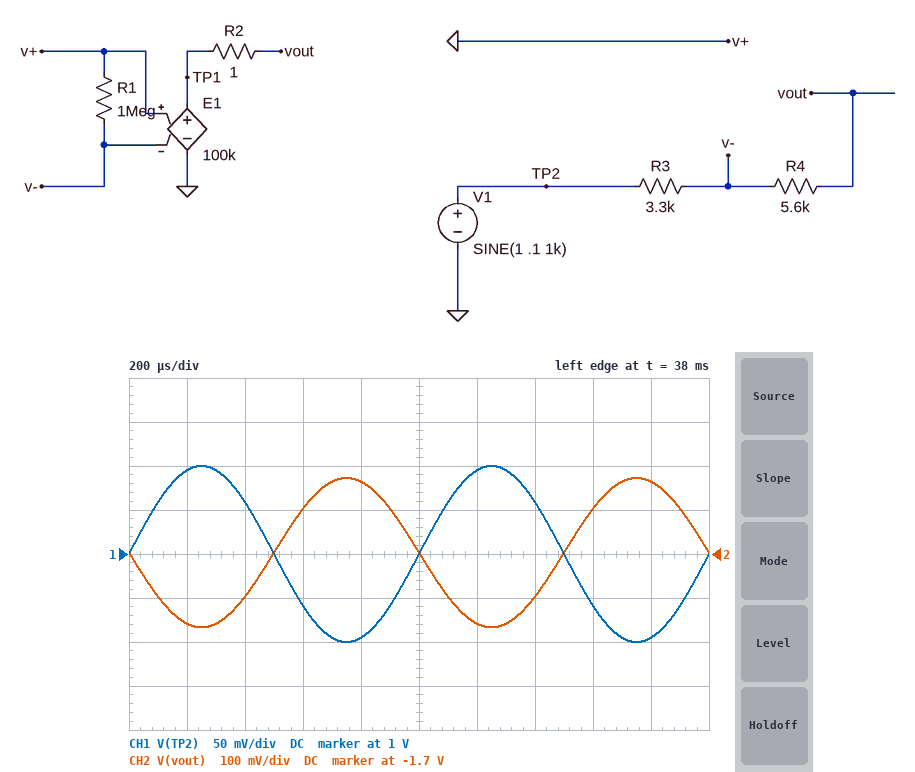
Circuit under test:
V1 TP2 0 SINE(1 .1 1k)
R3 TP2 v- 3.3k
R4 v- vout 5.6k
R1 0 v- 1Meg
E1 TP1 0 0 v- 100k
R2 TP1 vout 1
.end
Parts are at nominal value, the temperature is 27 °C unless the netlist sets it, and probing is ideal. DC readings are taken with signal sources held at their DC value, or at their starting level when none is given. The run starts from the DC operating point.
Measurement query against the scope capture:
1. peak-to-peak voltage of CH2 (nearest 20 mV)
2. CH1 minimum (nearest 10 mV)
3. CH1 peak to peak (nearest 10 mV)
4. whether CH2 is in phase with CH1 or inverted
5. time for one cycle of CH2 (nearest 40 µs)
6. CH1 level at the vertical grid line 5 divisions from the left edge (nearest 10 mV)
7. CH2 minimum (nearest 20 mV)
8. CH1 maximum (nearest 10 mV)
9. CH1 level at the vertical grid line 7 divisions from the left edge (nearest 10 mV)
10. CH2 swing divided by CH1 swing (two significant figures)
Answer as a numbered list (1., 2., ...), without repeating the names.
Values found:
1. 340 mV
2. 900 mV
3. 200 mV
4. inverted
5. 1.00 ms
6. 1.00 V
7. -1.86 V
8. 1.10 V
9. 1.06 V
10. 1.7
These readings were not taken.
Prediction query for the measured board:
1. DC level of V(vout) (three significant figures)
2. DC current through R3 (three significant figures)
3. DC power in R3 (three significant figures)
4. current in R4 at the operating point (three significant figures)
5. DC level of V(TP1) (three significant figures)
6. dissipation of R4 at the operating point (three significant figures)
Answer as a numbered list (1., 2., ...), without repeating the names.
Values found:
1. -1.70 V
2. 303 µA
3. 303 µW
4. 303 µA
5. -1.70 V
6. 514 µW
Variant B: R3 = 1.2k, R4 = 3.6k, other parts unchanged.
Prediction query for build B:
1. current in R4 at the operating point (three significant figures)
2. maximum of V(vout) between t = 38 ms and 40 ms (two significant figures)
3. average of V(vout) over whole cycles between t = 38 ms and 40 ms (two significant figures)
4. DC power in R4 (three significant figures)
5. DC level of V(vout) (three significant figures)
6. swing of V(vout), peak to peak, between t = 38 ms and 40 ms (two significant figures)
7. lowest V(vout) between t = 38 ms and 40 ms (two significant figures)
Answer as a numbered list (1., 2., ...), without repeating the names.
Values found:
1. 833 µA
2. -2.7 V
3. -3.0 V
4. 2.50 mW
5. -3.00 V
6. 600 mV
7. -3.3 V
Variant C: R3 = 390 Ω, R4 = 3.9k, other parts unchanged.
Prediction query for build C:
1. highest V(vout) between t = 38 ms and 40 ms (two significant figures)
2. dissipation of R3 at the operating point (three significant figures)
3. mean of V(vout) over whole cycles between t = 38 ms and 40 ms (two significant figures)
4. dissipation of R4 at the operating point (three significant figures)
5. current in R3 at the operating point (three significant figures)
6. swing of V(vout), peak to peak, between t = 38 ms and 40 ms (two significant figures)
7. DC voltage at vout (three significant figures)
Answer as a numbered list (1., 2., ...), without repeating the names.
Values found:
1. -9.0 V
2. 2.56 mW
3. -10 V
4. 25.6 mW
5. 2.56 mA
6. 2.0 V
7. -10.0 V
